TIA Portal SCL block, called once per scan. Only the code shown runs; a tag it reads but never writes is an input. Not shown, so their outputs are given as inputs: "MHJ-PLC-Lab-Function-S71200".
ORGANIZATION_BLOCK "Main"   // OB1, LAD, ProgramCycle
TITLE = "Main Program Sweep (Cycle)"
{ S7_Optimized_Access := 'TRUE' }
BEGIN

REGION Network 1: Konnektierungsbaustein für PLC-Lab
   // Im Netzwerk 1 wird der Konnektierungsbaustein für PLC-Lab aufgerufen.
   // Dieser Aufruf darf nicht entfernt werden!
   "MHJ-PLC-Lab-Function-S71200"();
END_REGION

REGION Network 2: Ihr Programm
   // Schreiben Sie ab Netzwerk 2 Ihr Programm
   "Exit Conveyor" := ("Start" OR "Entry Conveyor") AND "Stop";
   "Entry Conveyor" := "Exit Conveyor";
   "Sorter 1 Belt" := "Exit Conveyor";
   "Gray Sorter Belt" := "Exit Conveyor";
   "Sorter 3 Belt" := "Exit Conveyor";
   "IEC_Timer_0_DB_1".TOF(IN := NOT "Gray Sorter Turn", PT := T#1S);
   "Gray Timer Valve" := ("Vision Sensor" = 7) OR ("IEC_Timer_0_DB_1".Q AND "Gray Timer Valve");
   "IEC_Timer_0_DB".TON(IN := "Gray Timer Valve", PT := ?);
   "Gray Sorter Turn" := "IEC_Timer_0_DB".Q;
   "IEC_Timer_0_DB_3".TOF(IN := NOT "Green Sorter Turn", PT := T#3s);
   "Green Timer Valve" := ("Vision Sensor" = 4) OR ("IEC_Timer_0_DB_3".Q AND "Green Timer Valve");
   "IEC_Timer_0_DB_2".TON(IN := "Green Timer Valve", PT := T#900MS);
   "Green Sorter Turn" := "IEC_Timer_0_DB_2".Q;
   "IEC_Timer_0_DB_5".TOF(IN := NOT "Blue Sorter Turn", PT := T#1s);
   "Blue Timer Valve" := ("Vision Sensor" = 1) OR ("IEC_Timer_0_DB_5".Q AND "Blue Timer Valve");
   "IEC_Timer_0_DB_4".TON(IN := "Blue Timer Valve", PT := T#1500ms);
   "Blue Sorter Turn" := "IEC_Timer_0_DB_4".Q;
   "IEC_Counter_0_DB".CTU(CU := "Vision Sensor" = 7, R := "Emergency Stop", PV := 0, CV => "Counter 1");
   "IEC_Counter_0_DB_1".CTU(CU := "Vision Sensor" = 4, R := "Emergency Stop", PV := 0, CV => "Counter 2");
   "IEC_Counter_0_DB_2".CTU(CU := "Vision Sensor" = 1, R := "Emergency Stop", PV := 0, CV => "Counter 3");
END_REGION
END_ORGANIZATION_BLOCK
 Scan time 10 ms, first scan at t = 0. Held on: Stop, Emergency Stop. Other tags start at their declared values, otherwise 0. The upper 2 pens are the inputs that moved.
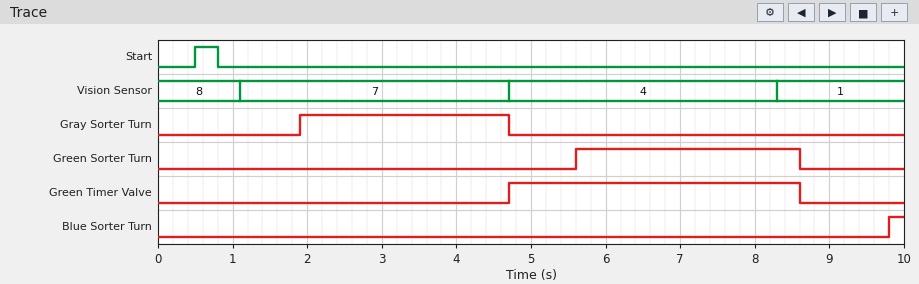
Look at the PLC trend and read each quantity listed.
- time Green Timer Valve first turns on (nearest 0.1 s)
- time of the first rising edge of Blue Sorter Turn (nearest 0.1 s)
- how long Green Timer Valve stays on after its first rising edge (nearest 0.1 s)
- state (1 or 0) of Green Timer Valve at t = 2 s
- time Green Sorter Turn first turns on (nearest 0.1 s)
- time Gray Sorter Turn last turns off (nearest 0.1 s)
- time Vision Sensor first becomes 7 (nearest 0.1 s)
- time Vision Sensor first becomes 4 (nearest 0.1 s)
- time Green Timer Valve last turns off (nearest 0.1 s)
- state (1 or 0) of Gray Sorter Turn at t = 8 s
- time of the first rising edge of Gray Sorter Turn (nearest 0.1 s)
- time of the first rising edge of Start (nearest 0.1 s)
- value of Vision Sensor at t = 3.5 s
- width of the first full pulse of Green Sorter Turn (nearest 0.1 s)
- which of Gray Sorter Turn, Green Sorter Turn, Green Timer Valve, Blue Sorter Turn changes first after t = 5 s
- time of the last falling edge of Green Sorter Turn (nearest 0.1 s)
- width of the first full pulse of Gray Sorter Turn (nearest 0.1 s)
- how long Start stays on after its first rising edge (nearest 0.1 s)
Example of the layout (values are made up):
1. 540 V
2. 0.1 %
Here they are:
1. 4.7 s
2. 9.8 s
3. 3.9 s
4. 0
5. 5.6 s
6. 4.7 s
7. 1.1 s
8. 4.7 s
9. 8.6 s
10. 0
11. 1.9 s
12. 0.5 s
13. 7
14. 3.0 s
15. Green Sorter Turn
16. 8.6 s
17. 2.8 s
18. 0.3 s
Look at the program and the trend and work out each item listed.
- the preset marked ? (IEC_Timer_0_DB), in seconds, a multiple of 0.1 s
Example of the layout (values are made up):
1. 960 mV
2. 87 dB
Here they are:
1. 0.8 s
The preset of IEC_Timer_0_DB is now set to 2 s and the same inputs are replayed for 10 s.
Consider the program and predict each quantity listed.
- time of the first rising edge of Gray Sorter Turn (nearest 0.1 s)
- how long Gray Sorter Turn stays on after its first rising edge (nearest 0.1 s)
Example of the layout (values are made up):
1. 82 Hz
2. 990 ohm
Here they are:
1. 3.1 s
2. 1.6 s
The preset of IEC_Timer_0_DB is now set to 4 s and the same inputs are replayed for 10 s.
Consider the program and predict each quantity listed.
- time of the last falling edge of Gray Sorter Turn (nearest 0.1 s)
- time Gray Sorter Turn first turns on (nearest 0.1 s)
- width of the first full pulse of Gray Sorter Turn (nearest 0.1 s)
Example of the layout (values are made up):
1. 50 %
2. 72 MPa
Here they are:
1. 6.1 s
2. 5.1 s
3. 1.0 s
